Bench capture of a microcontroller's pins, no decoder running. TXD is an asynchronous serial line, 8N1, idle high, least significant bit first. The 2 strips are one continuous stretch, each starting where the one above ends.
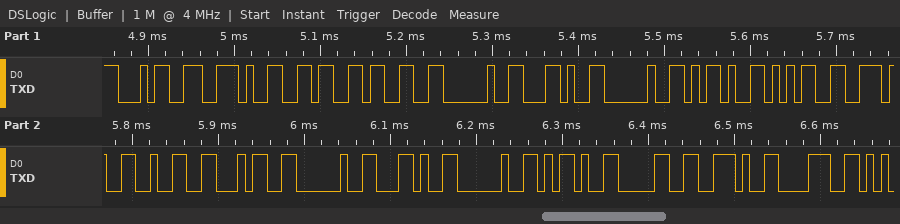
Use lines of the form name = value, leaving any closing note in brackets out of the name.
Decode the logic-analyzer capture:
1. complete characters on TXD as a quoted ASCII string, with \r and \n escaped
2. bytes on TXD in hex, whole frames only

complete characters on TXD as a quoted ASCII string, with \r and \n escaped = "4.63 , -5.24 , -0.8"
bytes on TXD in hex, whole frames only = 34 2E 36 33 20 2C 20 2D 35 2E 32 34 20 2C 20 2D 30 2E 38
